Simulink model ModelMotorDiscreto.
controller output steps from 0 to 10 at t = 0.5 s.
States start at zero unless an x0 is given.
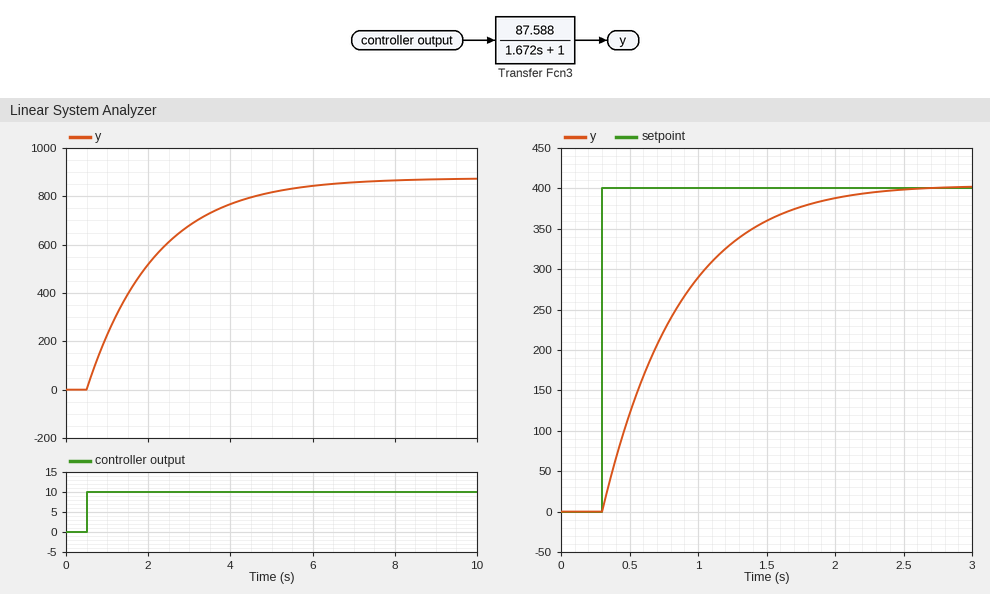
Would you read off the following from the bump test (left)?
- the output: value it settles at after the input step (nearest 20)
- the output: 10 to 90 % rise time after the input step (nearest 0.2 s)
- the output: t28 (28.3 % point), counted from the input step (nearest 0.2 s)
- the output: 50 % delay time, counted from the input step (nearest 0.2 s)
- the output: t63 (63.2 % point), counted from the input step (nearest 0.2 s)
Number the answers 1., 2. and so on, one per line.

1. 880
2. 3.6 s
3. 0.6 s
4. 1.2 s
5. 1.6 s
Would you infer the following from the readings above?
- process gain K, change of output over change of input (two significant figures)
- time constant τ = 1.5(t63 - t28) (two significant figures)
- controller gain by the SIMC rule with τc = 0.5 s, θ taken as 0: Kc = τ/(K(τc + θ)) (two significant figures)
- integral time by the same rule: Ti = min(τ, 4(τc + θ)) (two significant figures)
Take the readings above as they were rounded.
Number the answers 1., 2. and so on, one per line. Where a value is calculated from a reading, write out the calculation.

1. (880 - 0) / 10 = 88
2. 1.5 × (1.6 - 0.6) = 1.5 s
3. 1.5 / (88 × (0.5 + 0)) = 0.034
4. min(1.5, 4 × (0.5 + 0)) = 1.5 s
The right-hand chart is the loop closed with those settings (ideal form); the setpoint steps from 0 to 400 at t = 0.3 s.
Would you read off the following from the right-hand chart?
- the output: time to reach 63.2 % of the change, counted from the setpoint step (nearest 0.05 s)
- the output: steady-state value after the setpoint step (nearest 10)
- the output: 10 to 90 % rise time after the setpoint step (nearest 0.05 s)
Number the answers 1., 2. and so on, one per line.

1. 0.55 s
2. 400
3. 1.15 s
